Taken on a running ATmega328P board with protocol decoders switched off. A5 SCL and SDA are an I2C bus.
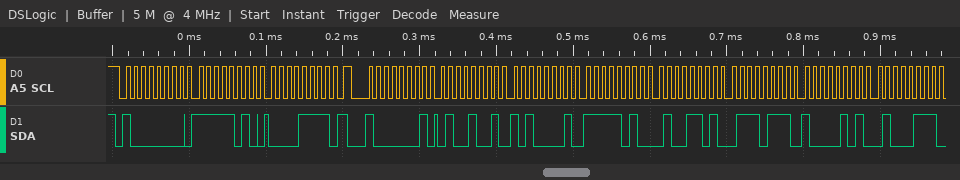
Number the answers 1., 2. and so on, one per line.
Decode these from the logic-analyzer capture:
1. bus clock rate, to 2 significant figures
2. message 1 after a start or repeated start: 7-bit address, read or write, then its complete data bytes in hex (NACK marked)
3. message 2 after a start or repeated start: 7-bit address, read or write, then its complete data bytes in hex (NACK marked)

1. 100 kHz
2. 0x40 write: FA 0F
3. 0x40 read: 49 A1 FA 4D 77 85 47
